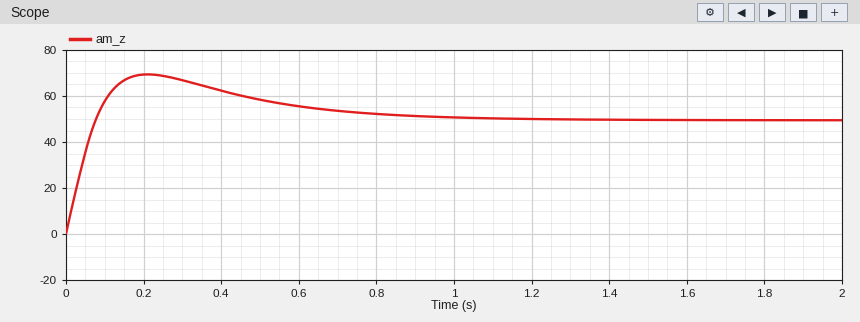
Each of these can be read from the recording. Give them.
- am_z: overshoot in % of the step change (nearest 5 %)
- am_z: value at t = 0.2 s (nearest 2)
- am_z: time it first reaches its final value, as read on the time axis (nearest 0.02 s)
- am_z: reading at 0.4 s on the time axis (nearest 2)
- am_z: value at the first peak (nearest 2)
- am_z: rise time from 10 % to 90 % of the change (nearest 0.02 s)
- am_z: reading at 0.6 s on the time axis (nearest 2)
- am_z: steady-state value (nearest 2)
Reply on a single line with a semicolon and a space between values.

40 %; 70; 0.08 s; 62; 70; 0.06 s; 56; 50
